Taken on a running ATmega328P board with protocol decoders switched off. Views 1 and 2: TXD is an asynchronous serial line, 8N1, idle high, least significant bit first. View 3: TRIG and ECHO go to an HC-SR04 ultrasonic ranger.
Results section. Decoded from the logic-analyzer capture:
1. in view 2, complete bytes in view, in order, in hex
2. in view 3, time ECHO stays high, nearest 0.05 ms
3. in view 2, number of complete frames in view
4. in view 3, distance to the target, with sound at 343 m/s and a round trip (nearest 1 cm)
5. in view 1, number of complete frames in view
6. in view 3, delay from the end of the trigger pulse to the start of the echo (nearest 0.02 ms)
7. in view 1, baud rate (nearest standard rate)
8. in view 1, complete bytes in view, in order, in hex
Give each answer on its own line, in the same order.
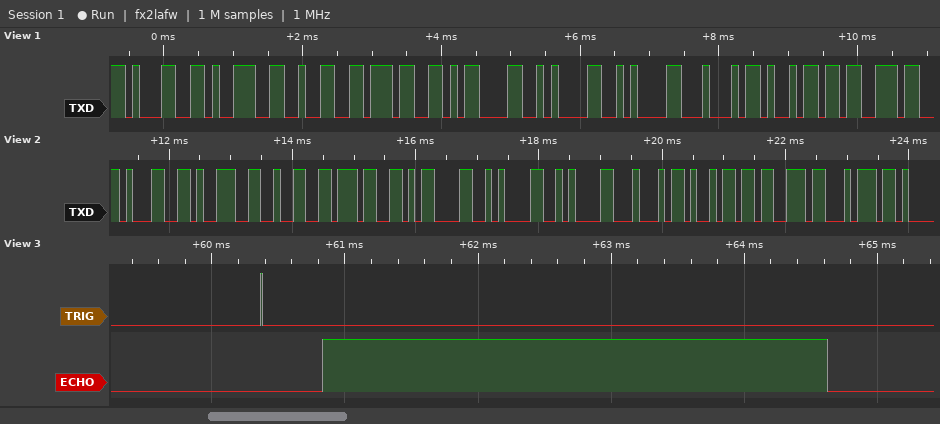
31 39 32 37 0D 0A 0A 44 69 73 74
3.80 ms
11
65 cm
10
0.46 ms
9600 baud
31 39 32 37 0D 0A 0A 44 69 73
